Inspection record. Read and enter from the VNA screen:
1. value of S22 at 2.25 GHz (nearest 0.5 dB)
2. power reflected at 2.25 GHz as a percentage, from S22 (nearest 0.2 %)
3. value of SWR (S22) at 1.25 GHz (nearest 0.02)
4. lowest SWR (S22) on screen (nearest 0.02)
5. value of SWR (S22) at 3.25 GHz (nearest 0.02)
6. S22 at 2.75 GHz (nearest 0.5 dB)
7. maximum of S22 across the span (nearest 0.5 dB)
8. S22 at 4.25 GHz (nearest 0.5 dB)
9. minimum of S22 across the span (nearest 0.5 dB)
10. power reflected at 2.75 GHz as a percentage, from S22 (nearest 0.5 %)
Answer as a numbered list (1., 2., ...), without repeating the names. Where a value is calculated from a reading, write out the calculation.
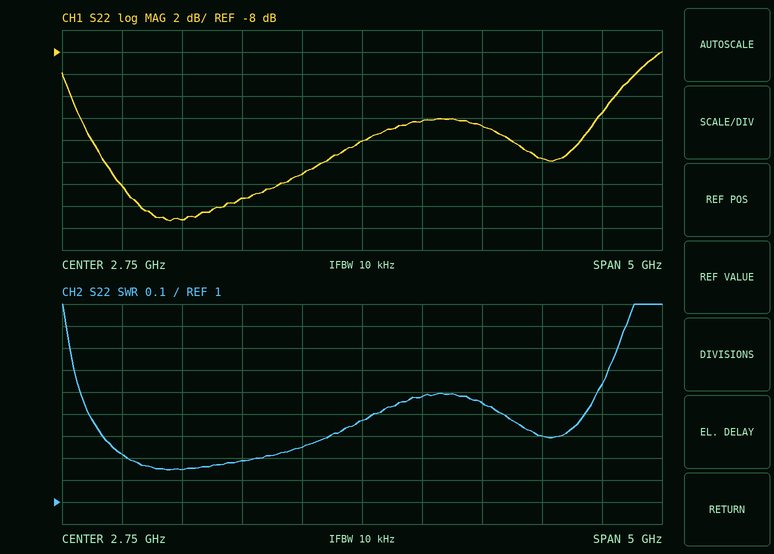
1. -19.0 dB
2. 10^(-19/10) ≈ 1.26 %, so 1.2 % to the nearest 0.2 %
3. 1.14
4. 1.14
5. 1.48
6. -16.0 dB
7. -8.0 dB
8. -17.5 dB
9. -23.5 dB
10. 10^(-16/10) ≈ 2.5 %
